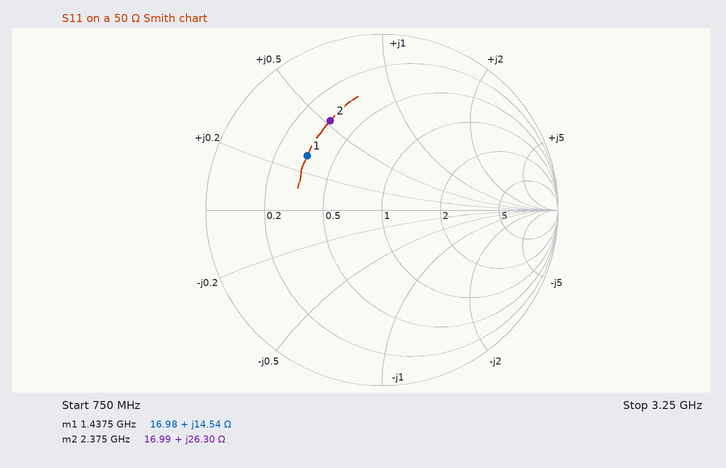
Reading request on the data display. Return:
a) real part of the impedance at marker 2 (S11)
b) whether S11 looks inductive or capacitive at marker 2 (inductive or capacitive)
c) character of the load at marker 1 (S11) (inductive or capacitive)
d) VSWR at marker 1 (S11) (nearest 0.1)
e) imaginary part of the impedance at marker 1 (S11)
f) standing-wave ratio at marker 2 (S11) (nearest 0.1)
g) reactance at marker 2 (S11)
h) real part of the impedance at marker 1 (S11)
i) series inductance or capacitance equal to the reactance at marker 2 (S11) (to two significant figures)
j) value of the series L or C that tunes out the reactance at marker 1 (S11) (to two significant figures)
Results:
16.99 Ω
inductive
inductive
3.2
+14.54 Ω
3.8
+26.30 Ω
16.98 Ω
1.8 nH
7.6 pF
